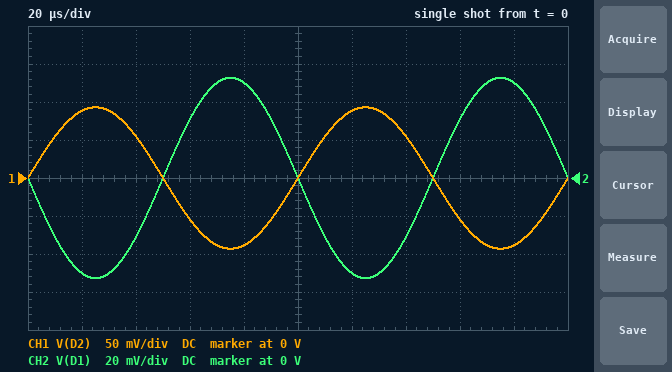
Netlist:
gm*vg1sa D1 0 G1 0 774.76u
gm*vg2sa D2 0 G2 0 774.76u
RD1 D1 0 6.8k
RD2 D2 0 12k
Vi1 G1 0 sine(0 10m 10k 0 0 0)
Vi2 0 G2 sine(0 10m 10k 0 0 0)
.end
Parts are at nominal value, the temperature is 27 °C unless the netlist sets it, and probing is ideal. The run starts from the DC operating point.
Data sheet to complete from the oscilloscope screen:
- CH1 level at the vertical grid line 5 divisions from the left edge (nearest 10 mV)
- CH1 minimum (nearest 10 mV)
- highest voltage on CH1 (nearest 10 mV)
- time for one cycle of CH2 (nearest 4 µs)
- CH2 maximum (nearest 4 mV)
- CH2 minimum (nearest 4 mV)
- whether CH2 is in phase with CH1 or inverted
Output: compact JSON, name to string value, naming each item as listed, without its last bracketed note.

{"CH1 level at the vertical grid line 5 divisions from the left edge": "0 V", "CH1 minimum": "-90 mV", "highest voltage on CH1": "90 mV", "time for one cycle of CH2": "100 µs", "CH2 maximum": "52 mV", "CH2 minimum": "-52 mV", "whether CH2 is in phase with CH1 or inverted": "inverted"}
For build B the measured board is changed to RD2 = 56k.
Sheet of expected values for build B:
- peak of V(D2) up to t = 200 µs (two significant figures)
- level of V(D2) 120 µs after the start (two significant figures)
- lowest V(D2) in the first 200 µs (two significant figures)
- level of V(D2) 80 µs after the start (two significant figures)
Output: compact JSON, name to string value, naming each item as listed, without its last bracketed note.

{"peak of V(D2) up to t = 200 µs": "430 mV", "level of V(D2) 120 µs after the start": "410 mV", "lowest V(D2) in the first 200 µs": "-430 mV", "level of V(D2) 80 µs after the start": "-410 mV"}
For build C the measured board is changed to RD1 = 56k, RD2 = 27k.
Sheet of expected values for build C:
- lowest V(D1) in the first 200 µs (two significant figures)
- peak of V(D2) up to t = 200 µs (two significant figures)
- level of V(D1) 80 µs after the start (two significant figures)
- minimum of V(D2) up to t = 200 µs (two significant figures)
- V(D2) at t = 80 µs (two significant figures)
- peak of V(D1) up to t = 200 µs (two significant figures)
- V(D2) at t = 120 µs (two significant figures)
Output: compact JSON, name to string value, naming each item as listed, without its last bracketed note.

{"lowest V(D1) in the first 200 µs": "-430 mV", "peak of V(D2) up to t = 200 µs": "210 mV", "level of V(D1) 80 µs after the start": "410 mV", "minimum of V(D2) up to t = 200 µs": "-210 mV", "V(D2) at t = 80 µs": "-200 mV", "peak of V(D1) up to t = 200 µs": "430 mV", "V(D2) at t = 120 µs": "200 mV"}
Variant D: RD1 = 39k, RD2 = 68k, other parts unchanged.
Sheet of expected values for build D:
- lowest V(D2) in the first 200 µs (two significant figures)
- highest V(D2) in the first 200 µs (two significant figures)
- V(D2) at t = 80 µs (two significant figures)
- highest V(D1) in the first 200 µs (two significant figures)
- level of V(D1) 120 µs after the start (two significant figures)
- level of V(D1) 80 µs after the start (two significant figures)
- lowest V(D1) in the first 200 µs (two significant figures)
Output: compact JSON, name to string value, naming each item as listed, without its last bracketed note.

{"lowest V(D2) in the first 200 µs": "-530 mV", "highest V(D2) in the first 200 µs": "530 mV", "V(D2) at t = 80 µs": "-500 mV", "highest V(D1) in the first 200 µs": "300 mV", "level of V(D1) 120 µs after the start": "-290 mV", "level of V(D1) 80 µs after the start": "290 mV", "lowest V(D1) in the first 200 µs": "-300 mV"}
